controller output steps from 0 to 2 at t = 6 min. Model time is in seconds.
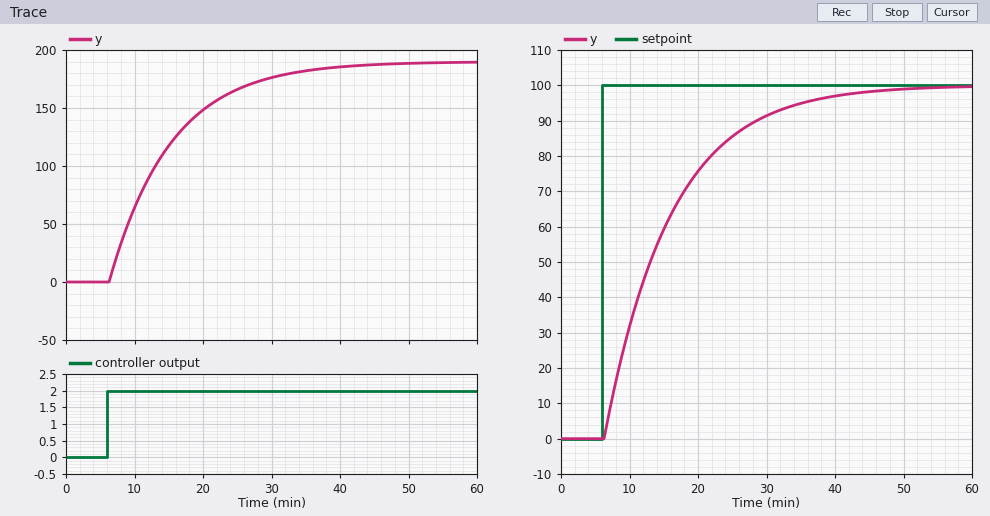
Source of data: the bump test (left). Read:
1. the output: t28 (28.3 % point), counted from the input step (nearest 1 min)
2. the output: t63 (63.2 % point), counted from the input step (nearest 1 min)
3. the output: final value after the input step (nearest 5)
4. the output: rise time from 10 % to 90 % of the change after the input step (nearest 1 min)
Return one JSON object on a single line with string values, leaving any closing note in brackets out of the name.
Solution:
{"the output: t28 (28.3 % point), counted from the input step": "3 min", "the output: t63 (63.2 % point), counted from the input step": "9 min", "the output: final value after the input step": "190", "the output: rise time from 10 % to 90 % of the change after the input step": "20 min"}
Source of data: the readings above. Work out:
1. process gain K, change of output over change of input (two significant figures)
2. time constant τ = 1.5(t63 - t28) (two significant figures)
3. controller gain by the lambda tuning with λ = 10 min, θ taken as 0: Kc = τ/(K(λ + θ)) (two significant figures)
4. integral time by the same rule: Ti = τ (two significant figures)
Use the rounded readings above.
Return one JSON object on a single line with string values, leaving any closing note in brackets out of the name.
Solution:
{"process gain K, change of output over change of input": "95", "time constant τ = 1.5(t63 - t28)": "9.0 min", "controller gain by the lambda tuning with λ = 10 min, θ taken as 0: Kc = τ/(K(λ + θ))": "0.0095", "integral time by the same rule: Ti = τ": "9.0 min"}
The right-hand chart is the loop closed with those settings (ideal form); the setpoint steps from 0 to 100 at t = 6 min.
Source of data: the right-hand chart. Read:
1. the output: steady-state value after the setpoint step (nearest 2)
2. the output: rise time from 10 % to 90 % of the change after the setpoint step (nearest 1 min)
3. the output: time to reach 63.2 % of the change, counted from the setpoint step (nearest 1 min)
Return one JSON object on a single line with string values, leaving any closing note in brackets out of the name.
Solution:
{"the output: steady-state value after the setpoint step": "100", "the output: rise time from 10 % to 90 % of the change after the setpoint step": "21 min", "the output: time to reach 63.2 % of the change, counted from the setpoint step": "10 min"}
